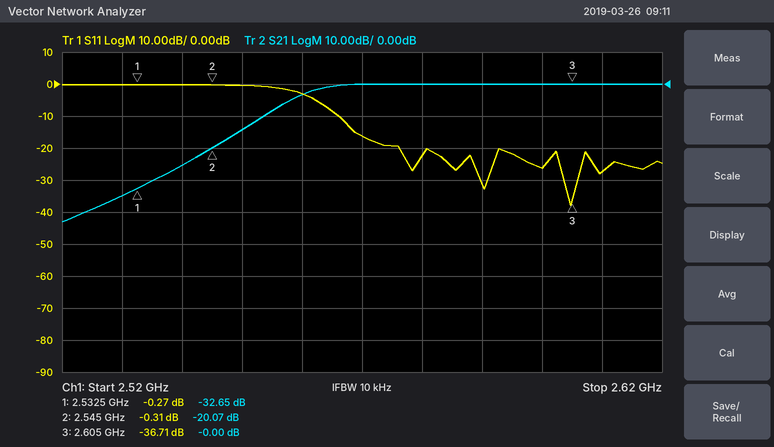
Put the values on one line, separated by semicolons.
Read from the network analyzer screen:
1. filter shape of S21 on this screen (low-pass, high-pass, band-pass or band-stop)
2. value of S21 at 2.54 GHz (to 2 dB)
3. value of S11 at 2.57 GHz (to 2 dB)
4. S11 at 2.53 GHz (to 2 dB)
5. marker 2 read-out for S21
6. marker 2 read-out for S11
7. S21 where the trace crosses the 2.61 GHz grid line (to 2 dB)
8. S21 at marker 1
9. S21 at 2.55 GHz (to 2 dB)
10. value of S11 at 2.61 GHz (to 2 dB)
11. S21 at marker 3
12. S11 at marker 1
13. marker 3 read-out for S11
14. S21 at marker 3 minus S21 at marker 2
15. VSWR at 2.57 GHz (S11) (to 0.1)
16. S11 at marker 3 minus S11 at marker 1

high-pass; -26 dB; -16 dB; 0 dB; -20.07 dB; -0.31 dB; 0 dB; -32.65 dB; -14 dB; -28 dB; -0.00 dB; -0.27 dB; -36.71 dB; 20.07 dB; 1.4; -36.44 dB
